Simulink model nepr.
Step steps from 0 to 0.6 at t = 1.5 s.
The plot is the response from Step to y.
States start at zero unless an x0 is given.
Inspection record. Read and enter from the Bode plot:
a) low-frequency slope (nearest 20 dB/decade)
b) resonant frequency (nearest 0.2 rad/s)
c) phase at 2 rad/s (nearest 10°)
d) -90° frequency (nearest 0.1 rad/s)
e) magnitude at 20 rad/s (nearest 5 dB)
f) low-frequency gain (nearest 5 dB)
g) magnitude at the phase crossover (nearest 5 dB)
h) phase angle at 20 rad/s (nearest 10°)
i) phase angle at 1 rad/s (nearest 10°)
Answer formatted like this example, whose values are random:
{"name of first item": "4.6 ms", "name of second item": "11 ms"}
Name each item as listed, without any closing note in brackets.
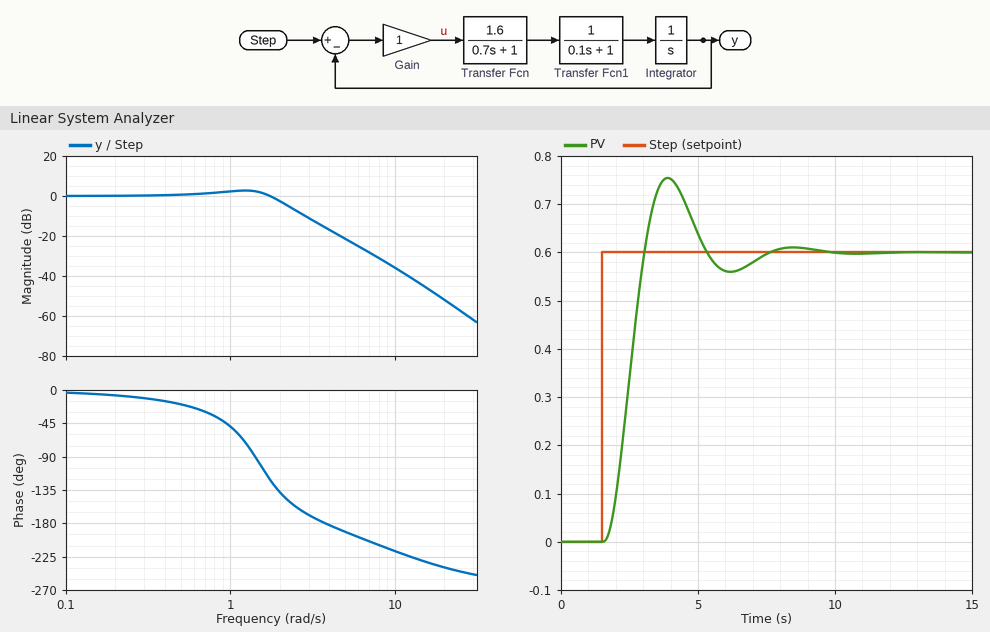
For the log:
{"low-frequency slope": "0 dB/decade", "resonant frequency": "1.2 rad/s", "phase at 2 rad/s": "-140°", "-90° frequency": "1.4 rad/s", "magnitude at 20 rad/s": "-50 dB", "low-frequency gain": "0 dB", "magnitude at the phase crossover": "-15 dB", "phase angle at 20 rad/s": "-240°", "phase angle at 1 rad/s": "-50°"}
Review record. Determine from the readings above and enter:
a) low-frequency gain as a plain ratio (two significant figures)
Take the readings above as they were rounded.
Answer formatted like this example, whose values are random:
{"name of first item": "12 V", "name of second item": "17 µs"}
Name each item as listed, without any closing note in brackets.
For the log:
{"low-frequency gain as a plain ratio": "1.0"}
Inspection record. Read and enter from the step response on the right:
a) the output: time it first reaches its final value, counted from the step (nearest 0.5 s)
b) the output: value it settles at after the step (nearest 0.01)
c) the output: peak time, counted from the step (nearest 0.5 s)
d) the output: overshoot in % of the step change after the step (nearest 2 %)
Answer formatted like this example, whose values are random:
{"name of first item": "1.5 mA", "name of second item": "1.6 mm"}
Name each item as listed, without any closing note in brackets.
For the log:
{"the output: time it first reaches its final value, counted from the step": "1.5 s", "the output: value it settles at after the step": "0.60", "the output: peak time, counted from the step": "2.5 s", "the output: overshoot in % of the step change after the step": "26 %"}
